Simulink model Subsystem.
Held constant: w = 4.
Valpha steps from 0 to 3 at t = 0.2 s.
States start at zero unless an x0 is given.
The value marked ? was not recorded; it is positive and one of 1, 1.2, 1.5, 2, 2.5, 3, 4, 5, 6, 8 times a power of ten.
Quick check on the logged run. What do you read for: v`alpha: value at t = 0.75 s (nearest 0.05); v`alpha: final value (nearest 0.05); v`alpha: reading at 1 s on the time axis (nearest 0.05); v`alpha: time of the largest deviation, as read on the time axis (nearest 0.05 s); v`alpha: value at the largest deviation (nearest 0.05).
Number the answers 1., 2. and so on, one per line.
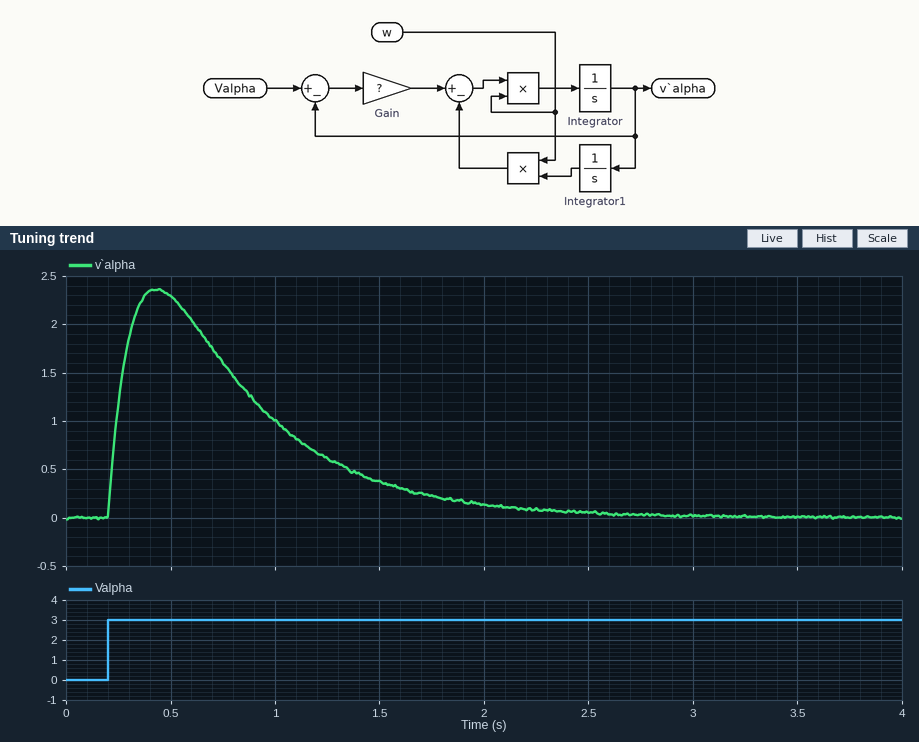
1. 1.60
2. 0.00
3. 1.00
4. 0.45 s
5. 2.35
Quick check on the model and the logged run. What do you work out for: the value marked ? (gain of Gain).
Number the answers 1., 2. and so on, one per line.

1. 2.5
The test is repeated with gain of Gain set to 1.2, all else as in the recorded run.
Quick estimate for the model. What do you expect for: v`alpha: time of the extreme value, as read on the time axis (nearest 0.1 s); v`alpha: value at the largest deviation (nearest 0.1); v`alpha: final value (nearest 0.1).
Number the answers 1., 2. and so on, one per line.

1. 0.5 s
2. 1.8
3. 0.0
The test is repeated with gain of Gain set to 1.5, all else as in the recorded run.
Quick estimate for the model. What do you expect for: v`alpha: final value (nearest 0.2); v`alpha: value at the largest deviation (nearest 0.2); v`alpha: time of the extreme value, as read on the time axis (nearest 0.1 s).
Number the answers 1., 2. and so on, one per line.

1. 0.0
2. 2.0
3. 0.5 s
